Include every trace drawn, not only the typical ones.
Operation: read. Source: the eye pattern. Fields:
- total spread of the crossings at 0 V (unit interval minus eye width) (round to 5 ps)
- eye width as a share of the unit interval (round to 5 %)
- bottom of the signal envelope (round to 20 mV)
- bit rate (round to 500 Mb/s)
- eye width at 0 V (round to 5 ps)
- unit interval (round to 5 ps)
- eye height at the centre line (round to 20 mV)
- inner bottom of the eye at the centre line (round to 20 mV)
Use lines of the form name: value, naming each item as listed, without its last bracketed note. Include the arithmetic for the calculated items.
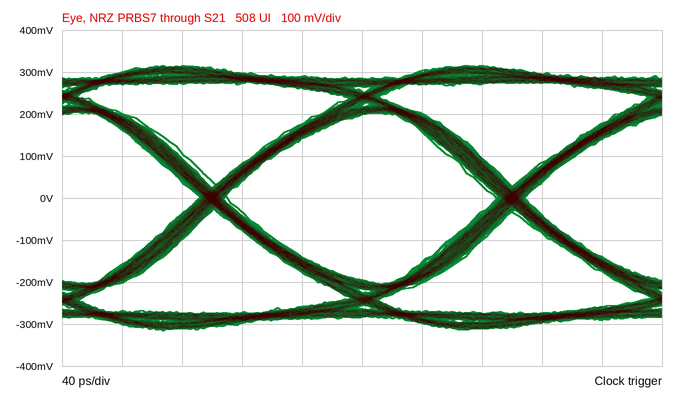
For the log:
total spread of the crossings at 0 V (unit interval minus eye width): 20 ps
eye width as a share of the unit interval: 180 ps / 200 ps ≈ 90 %
bottom of the signal envelope: -320 mV
bit rate: 5.0 Gb/s
eye width at 0 V: 180 ps
unit interval: 200 ps
eye height at the centre line: 400 mV
inner bottom of the eye at the centre line: -200 mV
